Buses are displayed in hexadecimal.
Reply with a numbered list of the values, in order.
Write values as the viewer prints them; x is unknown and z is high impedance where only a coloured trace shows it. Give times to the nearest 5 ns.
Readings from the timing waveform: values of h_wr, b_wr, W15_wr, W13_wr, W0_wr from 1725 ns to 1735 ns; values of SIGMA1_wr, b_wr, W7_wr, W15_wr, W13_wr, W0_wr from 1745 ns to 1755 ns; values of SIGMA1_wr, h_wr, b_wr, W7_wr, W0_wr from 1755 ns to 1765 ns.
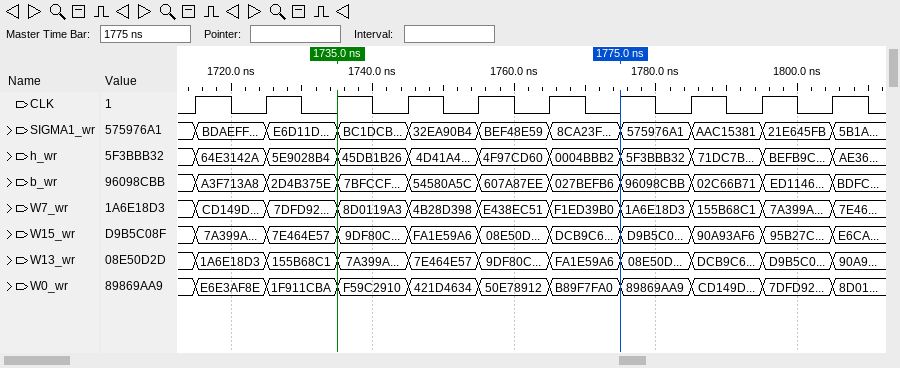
1. h_wr=5E9028B4, b_wr=2D4B375E, W15_wr=7E464E57, W13_wr=155B68C1, W0_wr=1F911CBA
2. SIGMA1_wr=32EA90B4, b_wr=54580A5C, W7_wr=4B28D398, W15_wr=FA1E59A6, W13_wr=7E464E57, W0_wr=421D4634
3. SIGMA1_wr=BEF48E59, h_wr=4F97CD60, b_wr=607A87EE, W7_wr=E438EC51, W0_wr=50E78912
